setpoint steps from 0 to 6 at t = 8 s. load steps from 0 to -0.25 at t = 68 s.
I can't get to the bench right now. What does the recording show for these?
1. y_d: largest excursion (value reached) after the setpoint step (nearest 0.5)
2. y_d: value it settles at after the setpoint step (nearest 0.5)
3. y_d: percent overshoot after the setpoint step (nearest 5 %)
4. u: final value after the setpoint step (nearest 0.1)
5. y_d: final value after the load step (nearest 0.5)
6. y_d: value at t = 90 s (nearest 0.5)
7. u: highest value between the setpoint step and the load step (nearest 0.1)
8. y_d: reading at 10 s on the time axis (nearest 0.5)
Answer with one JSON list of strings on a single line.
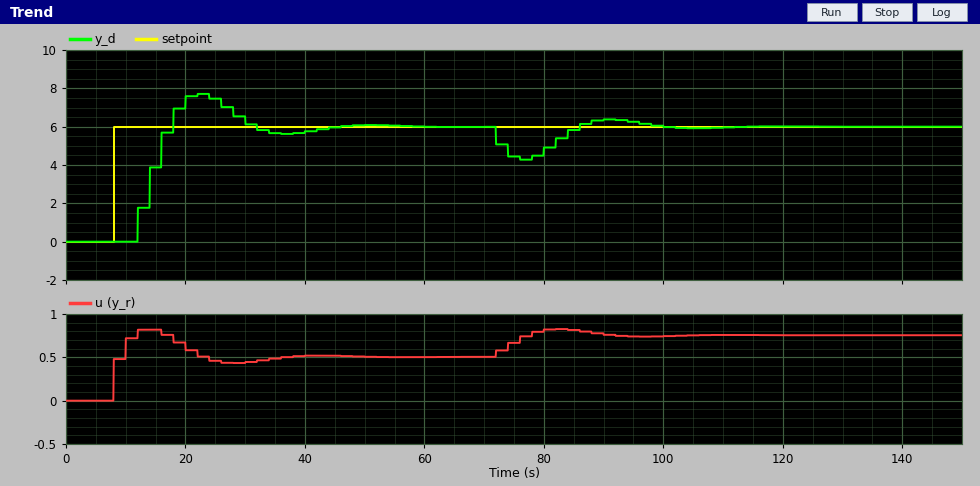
["7.5", "6.0", "30 %", "0.5", "6.0", "6.5", "0.8", "0.0"]
